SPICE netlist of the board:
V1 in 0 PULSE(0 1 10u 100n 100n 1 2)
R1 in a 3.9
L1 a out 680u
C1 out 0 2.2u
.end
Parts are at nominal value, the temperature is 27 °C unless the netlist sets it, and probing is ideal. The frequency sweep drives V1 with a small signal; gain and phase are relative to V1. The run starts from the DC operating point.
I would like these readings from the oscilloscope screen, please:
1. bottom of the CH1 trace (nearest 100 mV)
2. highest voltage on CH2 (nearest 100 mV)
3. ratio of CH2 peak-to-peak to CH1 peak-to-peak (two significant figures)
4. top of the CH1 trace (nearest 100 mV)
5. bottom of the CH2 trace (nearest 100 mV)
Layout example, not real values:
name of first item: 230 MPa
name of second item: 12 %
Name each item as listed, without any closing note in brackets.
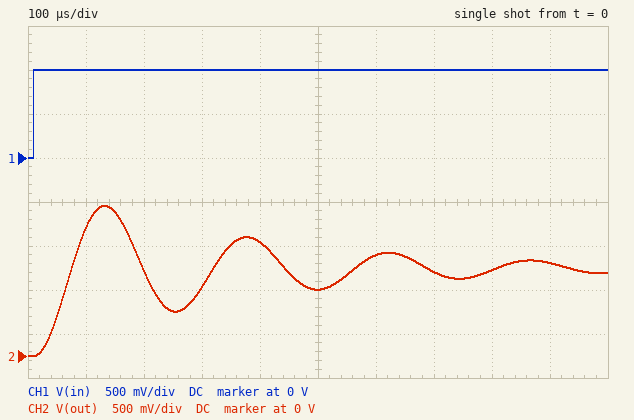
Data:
bottom of the CH1 trace: 0 V
highest voltage on CH2: 1.7 V
ratio of CH2 peak-to-peak to CH1 peak-to-peak: 1.7
top of the CH1 trace: 1.0 V
bottom of the CH2 trace: 0 V
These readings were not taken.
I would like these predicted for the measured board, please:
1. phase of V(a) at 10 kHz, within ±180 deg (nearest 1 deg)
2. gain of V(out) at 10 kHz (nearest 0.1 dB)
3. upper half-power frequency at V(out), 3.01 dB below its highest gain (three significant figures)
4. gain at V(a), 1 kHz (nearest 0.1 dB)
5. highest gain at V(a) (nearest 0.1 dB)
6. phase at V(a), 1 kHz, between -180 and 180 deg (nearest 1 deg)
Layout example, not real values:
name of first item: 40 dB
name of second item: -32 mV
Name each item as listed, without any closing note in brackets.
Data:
phase of V(a) at 10 kHz, within ±180 deg: 6 deg
gain of V(out) at 10 kHz: -13.9 dB
upper half-power frequency at V(out), 3.01 dB below its highest gain: 4.50 kHz
gain at V(a), 1 kHz: 0 dB
highest gain at V(a): 0 dB
phase at V(a), 1 kHz, between -180 and 180 deg: -3 deg
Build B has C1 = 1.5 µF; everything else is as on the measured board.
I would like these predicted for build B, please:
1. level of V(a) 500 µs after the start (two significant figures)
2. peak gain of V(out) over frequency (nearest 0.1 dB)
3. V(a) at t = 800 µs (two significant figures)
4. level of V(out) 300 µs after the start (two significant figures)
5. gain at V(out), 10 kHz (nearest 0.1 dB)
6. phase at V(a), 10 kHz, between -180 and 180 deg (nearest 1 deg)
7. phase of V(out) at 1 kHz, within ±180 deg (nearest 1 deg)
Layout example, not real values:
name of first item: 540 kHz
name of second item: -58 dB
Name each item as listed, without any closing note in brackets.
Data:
level of V(a) 500 µs after the start: 980 mV
peak gain of V(out) over frequency: 14.8 dB
V(a) at t = 800 µs: 1.0 V
level of V(out) 300 µs after the start: 1.4 V
gain at V(out), 10 kHz: -9.7 dB
phase at V(a), 10 kHz, between -180 and 180 deg: 7 deg
phase of V(out) at 1 kHz, within ±180 deg: -2 deg
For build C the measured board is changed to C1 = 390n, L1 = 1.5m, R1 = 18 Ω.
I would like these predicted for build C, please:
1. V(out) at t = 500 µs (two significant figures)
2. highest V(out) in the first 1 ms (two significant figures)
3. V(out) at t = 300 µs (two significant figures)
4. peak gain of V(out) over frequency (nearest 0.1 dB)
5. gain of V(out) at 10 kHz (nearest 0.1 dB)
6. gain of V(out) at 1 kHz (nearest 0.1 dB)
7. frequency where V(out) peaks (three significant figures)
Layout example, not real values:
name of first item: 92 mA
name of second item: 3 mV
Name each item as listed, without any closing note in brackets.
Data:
V(out) at t = 500 µs: 970 mV
highest V(out) in the first 1 ms: 1.6 V
V(out) at t = 300 µs: 880 mV
peak gain of V(out) over frequency: 10.8 dB
gain of V(out) at 10 kHz: -2.8 dB
gain of V(out) at 1 kHz: 0.2 dB
frequency where V(out) peaks: 6.44 kHz
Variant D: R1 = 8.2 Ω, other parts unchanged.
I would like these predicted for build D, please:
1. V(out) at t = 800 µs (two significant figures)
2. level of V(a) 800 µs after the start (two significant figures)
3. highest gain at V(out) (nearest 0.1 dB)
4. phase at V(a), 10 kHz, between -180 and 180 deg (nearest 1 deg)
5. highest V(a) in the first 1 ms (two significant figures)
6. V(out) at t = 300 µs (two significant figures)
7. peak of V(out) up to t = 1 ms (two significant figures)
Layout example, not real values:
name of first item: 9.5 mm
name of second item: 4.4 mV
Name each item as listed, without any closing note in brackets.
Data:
V(out) at t = 800 µs: 990 mV
level of V(a) 800 µs after the start: 1.0 V
highest gain at V(out): 6.9 dB
phase at V(a), 10 kHz, between -180 and 180 deg: 13 deg
highest V(a) in the first 1 ms: 1.2 V
V(out) at t = 300 µs: 870 mV
peak of V(out) up to t = 1 ms: 1.5 V
